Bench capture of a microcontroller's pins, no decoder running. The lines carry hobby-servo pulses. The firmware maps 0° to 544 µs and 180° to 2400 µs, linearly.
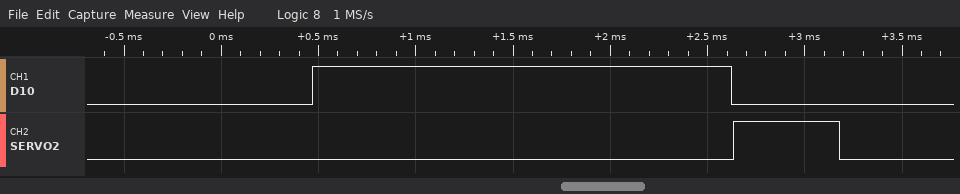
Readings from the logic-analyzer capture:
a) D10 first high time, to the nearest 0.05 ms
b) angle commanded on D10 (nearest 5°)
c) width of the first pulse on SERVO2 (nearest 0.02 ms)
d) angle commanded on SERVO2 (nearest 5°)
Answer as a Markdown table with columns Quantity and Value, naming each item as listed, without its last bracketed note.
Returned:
| Quantity | Value |
|---|---|
| D10 first high time, to the nearest 0.05 ms | 2.15 ms |
| angle commanded on D10 | 155° |
| width of the first pulse on SERVO2 | 0.54 ms |
| angle commanded on SERVO2 | 0° |
